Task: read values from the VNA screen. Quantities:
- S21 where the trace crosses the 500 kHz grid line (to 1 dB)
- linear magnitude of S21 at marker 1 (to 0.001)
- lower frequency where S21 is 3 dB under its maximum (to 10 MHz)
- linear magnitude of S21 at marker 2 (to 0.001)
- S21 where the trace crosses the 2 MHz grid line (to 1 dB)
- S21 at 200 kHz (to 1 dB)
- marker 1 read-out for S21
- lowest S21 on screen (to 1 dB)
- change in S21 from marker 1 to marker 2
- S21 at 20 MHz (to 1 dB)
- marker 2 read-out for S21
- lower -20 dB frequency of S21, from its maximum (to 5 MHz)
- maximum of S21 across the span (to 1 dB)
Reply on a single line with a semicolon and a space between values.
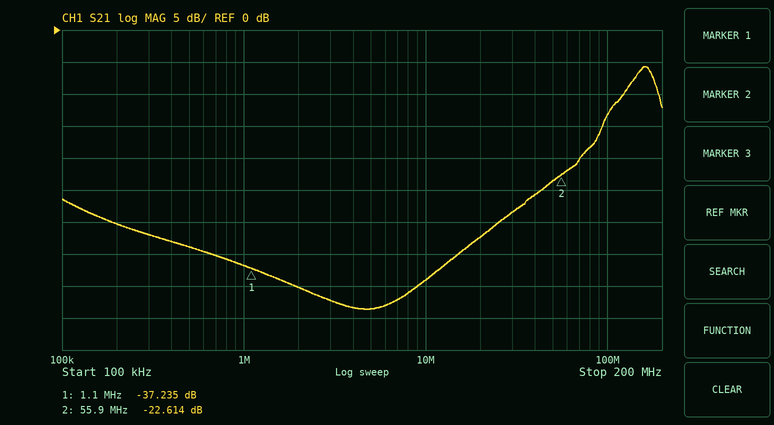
-34 dB; 0.014; 130 MHz; 0.074; -40 dB; -30 dB; -37.235 dB; -44 dB; 14.621 dB; -32 dB; -22.614 dB; 40 MHz; -6 dB
